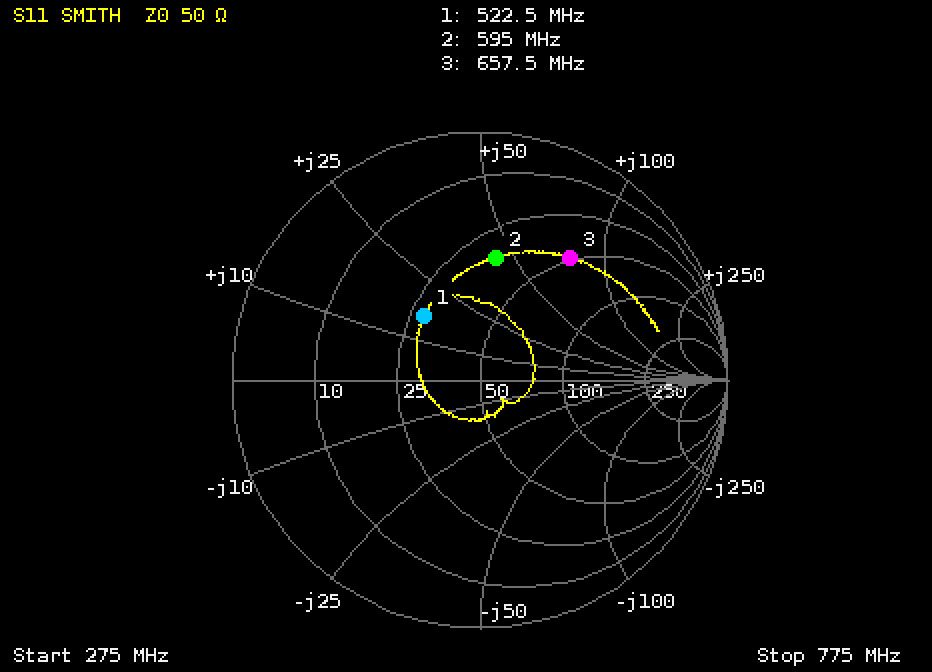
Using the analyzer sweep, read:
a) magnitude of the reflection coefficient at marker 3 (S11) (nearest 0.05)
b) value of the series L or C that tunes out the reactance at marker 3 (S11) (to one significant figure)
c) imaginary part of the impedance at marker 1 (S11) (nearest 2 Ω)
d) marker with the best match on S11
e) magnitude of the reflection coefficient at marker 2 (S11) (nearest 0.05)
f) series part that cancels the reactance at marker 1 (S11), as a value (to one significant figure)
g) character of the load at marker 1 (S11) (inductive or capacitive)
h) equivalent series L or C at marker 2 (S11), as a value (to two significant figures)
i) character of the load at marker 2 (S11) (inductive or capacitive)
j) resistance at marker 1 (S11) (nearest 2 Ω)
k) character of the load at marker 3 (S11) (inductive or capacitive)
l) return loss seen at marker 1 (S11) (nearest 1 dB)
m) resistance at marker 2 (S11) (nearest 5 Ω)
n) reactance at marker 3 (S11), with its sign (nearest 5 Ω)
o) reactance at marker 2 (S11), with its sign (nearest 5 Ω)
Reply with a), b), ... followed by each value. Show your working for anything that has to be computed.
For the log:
a) 0.60
b) C = 1/(2π × 657.5 MHz × 75 Ω) ≈ 3 pF
c) +16 Ω
d) marker 1
e) 0.50
f) C = 1/(2π × 522.5 MHz × 16 Ω) ≈ 19.0 pF, so 20 pF to one significant figure
g) inductive
h) L = 45 Ω/(2π × 595 MHz) ≈ 12 nH
i) inductive
j) 28 Ω
k) inductive
l) 9 dB
m) 35 Ω
n) +75 Ω
o) +45 Ω
